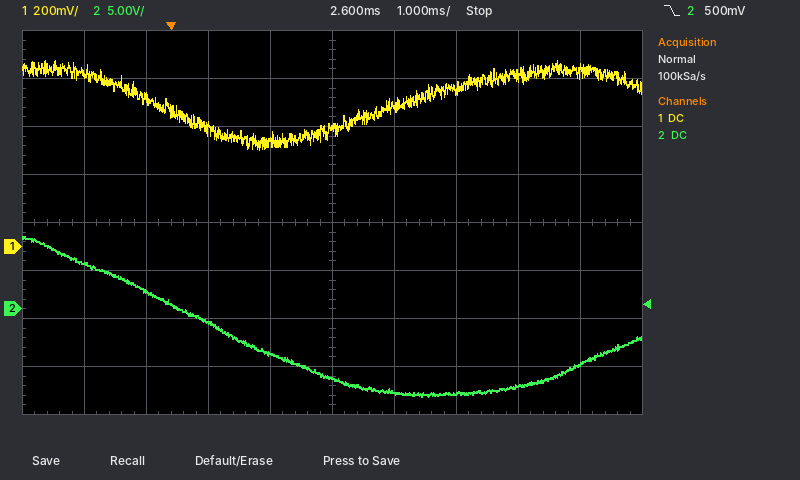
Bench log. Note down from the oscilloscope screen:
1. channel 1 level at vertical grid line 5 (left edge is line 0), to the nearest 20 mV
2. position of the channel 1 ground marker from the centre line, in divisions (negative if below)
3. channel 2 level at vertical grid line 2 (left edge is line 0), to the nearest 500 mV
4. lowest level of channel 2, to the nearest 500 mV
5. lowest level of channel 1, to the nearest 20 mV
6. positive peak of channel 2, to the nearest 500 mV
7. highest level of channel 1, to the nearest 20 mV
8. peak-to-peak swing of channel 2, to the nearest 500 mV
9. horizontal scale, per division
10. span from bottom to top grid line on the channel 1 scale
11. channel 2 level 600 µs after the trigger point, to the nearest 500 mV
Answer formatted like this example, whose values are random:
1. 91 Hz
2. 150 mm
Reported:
1. 500 mV
2. -0.5 div
3. 2.0 V
4. -9.0 V
5. 400 mV
6. 7.5 V
7. 780 mV
8. 16.5 V
9. 1 ms
10. 1.6 V
11. -1.5 V
